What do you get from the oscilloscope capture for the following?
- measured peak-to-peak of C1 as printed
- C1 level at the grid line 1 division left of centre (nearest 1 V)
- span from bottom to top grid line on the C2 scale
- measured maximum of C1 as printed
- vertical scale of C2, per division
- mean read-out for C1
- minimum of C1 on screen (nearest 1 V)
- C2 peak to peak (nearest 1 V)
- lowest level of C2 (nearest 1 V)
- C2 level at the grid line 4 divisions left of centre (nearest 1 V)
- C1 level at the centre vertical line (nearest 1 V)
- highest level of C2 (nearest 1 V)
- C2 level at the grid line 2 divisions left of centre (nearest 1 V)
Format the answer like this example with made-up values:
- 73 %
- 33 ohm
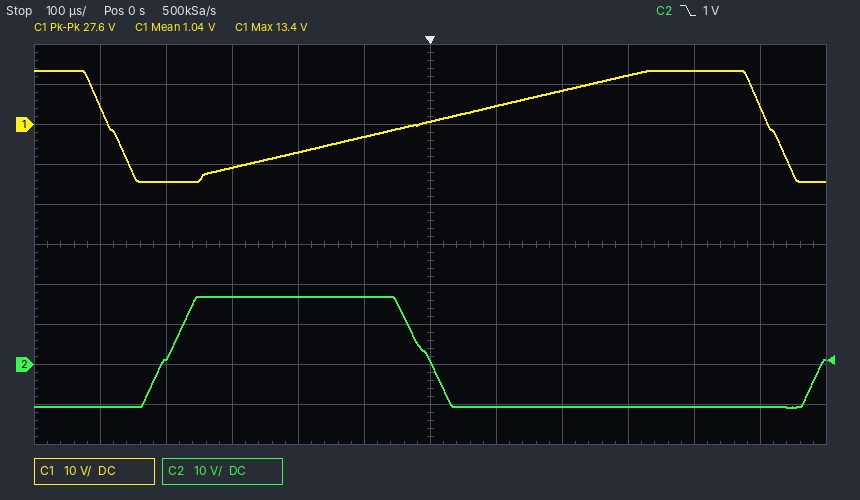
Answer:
- 27.6 V
- -3 V
- 100 V
- 13.4 V
- 10 V
- 1.04 V
- -14 V
- 28 V
- -11 V
- 2 V
- 1 V
- 17 V
- 17 V
